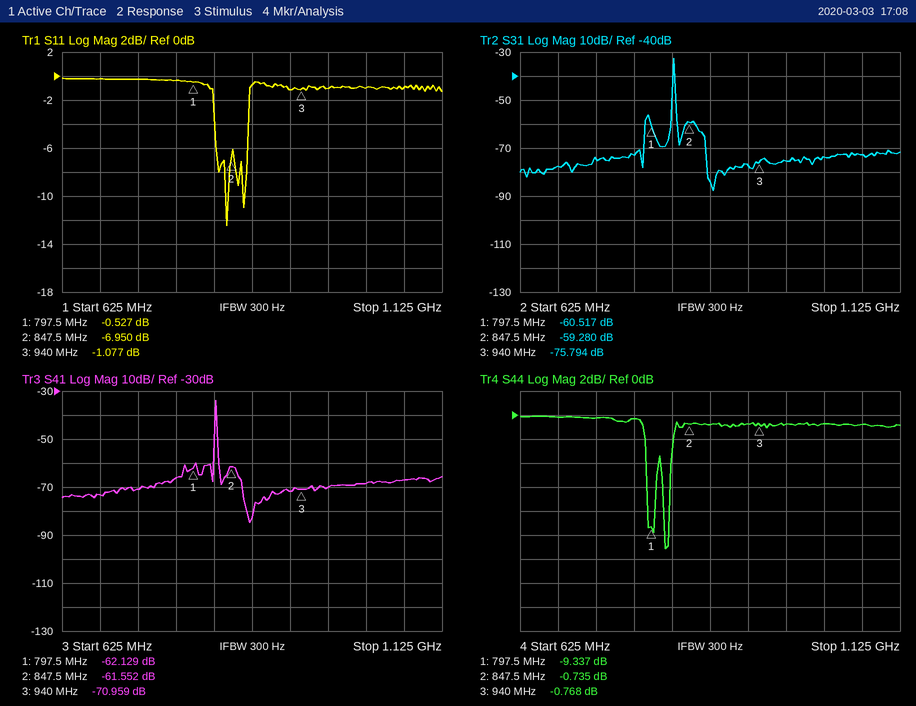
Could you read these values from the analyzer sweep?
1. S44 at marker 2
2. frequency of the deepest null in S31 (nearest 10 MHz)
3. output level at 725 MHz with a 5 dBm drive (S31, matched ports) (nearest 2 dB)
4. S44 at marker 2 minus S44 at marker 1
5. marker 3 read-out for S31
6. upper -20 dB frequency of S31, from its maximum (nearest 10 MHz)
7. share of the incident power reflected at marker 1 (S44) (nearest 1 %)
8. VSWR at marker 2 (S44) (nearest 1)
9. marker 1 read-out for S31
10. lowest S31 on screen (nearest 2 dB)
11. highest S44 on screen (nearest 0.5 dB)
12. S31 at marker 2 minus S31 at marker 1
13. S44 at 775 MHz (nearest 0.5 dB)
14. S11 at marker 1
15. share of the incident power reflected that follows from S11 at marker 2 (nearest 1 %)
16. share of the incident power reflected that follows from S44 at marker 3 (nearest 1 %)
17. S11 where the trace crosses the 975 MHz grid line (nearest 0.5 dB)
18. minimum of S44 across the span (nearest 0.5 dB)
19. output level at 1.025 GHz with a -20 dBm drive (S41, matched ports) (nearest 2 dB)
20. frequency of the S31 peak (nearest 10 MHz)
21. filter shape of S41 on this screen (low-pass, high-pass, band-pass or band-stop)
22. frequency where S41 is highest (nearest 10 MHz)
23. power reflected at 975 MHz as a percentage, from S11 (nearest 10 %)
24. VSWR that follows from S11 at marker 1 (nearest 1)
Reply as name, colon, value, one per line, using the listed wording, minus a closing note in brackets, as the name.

S44 at marker 2: -0.735 dB
frequency of the deepest null in S31: 880 MHz
output level at 725 MHz with a 5 dBm drive (S31, matched ports): -70 dBm
S44 at marker 2 minus S44 at marker 1: 8.602 dB
marker 3 read-out for S31: -75.794 dB
upper -20 dB frequency of S31, from its maximum: 830 MHz
share of the incident power reflected at marker 1 (S44): 12 %
VSWR at marker 2 (S44): 24
marker 1 read-out for S31: -60.517 dB
lowest S31 on screen: -88 dB
highest S44 on screen: 0.0 dB
S31 at marker 2 minus S31 at marker 1: 1.237 dB
S44 at 775 MHz: -0.5 dB
S11 at marker 1: -0.527 dB
share of the incident power reflected that follows from S11 at marker 2: 20 %
share of the incident power reflected that follows from S44 at marker 3: 84 %
S11 where the trace crosses the 975 MHz grid line: -1.0 dB
minimum of S44 across the span: -11.0 dB
output level at 1.025 GHz with a -20 dBm drive (S41, matched ports): -88 dBm
frequency of the S31 peak: 830 MHz
filter shape of S41 on this screen: band-pass
frequency where S41 is highest: 830 MHz
power reflected at 975 MHz as a percentage, from S11: 80 %
VSWR that follows from S11 at marker 1: 33
